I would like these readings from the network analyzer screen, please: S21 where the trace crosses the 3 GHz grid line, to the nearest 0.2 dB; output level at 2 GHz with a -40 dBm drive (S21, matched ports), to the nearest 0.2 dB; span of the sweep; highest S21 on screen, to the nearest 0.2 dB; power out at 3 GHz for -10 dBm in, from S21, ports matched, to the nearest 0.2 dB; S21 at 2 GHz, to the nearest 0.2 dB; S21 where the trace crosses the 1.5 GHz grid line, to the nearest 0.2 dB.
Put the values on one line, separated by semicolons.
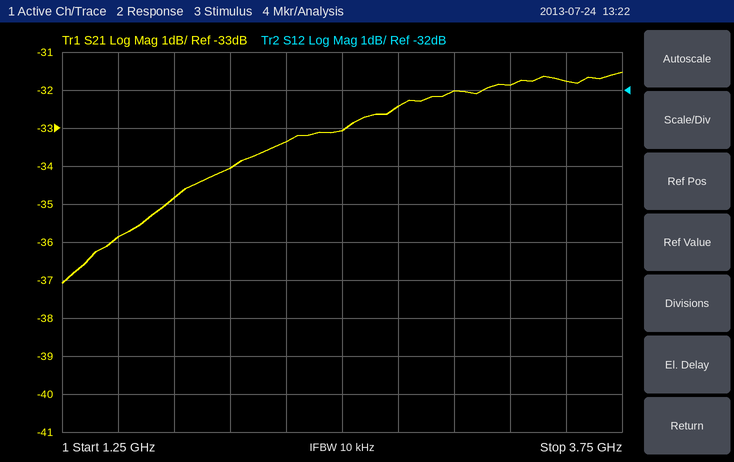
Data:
-32.0 dB; -74.0 dBm; 2.5 GHz; -31.6 dB; -42.0 dBm; -34.0 dB; -35.8 dB
